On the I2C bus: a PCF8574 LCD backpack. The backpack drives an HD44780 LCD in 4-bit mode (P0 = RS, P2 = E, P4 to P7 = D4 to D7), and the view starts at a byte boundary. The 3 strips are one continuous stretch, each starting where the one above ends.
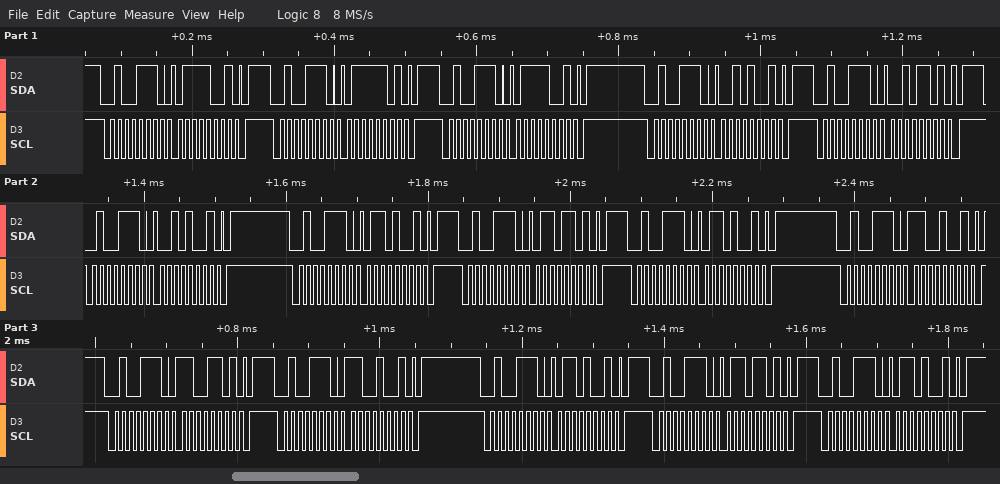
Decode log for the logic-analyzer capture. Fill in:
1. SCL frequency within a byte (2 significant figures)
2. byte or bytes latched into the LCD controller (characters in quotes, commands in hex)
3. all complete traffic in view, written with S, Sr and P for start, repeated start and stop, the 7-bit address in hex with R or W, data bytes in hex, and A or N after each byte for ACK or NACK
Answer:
100 kHz
'r' 'l'
S 27W A 79 A P S 27W A 7D A P S 27W A 79 A P S 27W A 29 A P S 27W A 2D A P S 27W A 29 A P S 27W A 69 A P S 27W A 6D A P S 27W A 69 A P S 27W A C9 A P S 27W A CD A P S 27W A C9 A P S 27W A 69 A P S 27W A 6D A P S 27W A 69 A P
